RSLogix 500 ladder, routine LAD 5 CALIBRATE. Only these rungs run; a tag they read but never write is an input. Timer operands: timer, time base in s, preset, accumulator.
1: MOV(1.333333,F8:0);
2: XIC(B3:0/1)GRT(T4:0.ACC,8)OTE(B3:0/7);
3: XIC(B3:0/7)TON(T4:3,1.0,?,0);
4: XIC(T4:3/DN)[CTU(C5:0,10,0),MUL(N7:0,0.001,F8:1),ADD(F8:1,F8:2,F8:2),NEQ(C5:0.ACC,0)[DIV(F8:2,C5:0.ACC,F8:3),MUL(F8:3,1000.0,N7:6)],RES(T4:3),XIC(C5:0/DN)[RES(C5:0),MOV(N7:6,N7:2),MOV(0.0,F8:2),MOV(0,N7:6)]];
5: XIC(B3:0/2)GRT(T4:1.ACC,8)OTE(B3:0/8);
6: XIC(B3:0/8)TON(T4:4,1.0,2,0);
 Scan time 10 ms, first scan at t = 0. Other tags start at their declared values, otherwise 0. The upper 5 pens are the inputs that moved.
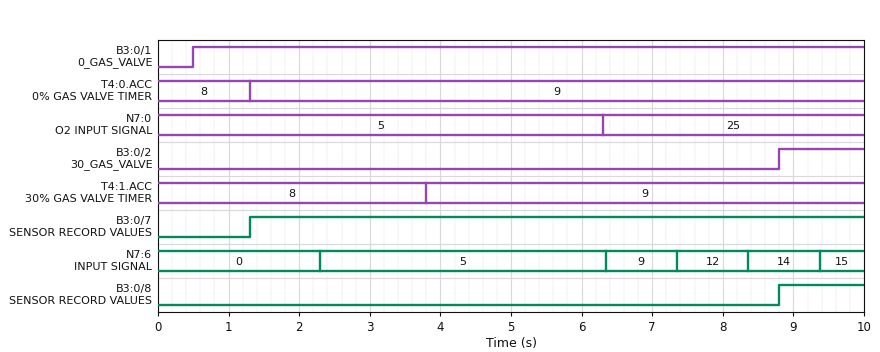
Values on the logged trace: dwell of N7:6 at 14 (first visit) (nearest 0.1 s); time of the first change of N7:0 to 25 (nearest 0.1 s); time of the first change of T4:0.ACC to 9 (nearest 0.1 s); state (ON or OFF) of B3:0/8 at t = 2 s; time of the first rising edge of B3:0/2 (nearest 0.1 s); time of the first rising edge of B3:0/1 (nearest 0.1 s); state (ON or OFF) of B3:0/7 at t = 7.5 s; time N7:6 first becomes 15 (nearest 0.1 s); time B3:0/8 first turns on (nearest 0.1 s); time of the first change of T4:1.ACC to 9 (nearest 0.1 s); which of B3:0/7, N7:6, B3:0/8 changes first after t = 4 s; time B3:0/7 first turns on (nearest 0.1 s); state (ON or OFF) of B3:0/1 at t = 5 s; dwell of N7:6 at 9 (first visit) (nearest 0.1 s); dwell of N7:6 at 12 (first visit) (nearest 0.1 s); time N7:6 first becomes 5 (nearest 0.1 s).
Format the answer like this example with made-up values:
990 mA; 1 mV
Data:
1.0 s; 6.3 s; 1.3 s; OFF; 8.8 s; 0.5 s; ON; 9.4 s; 8.8 s; 3.8 s; N7:6; 1.3 s; ON; 1.0 s; 1.0 s; 2.3 s
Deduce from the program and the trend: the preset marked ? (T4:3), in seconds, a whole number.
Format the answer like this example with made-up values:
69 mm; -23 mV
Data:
1 s
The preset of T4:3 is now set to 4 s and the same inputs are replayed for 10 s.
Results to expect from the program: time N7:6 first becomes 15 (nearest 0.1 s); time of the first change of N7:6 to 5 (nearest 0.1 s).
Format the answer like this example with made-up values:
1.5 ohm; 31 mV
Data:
9.3 s; 5.3 s
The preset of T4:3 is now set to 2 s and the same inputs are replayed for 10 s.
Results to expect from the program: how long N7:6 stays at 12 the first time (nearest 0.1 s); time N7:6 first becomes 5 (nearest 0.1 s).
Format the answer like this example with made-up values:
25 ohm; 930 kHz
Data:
2.0 s; 3.3 s
